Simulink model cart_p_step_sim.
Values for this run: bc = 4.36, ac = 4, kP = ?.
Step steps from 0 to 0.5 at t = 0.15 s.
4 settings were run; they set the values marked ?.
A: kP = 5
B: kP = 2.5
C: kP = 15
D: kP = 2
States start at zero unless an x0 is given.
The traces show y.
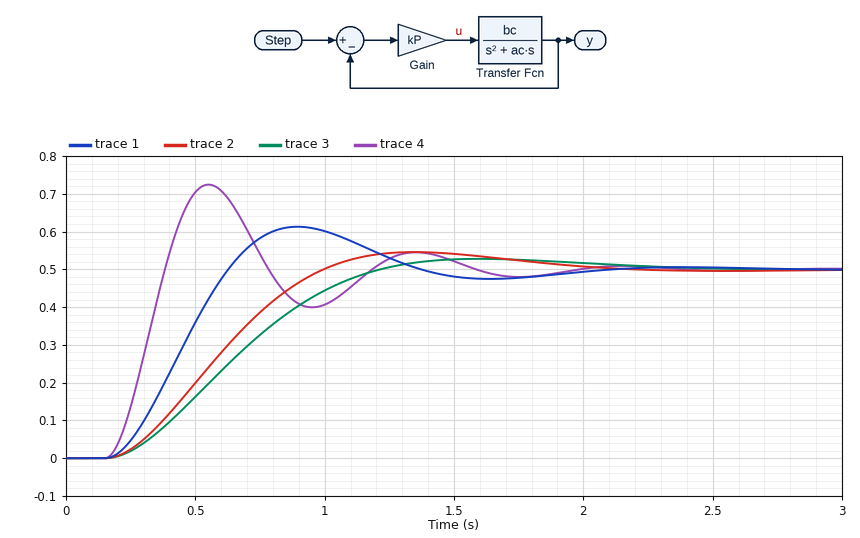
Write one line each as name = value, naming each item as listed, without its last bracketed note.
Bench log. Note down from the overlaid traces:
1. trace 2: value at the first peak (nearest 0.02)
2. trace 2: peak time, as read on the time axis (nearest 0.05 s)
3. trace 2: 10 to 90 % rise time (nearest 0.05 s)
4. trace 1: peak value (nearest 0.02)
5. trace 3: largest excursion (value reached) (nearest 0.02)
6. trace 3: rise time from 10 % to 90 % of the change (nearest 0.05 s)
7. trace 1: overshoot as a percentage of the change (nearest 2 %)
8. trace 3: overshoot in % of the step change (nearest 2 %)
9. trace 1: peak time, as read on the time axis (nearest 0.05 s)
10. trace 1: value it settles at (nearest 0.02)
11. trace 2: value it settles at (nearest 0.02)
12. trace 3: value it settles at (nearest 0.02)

trace 2: value at the first peak = 0.54
trace 2: peak time, as read on the time axis = 1.35 s
trace 2: 10 to 90 % rise time = 0.55 s
trace 1: peak value = 0.62
trace 3: largest excursion (value reached) = 0.52
trace 3: rise time from 10 % to 90 % of the change = 0.70 s
trace 1: overshoot as a percentage of the change = 22 %
trace 3: overshoot in % of the step change = 6 %
trace 1: peak time, as read on the time axis = 0.90 s
trace 1: value it settles at = 0.50
trace 2: value it settles at = 0.50
trace 3: value it settles at = 0.50
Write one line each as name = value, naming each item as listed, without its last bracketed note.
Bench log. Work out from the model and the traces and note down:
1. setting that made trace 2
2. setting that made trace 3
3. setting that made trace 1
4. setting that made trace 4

setting that made trace 2 = B
setting that made trace 3 = D
setting that made trace 1 = A
setting that made trace 4 = C
